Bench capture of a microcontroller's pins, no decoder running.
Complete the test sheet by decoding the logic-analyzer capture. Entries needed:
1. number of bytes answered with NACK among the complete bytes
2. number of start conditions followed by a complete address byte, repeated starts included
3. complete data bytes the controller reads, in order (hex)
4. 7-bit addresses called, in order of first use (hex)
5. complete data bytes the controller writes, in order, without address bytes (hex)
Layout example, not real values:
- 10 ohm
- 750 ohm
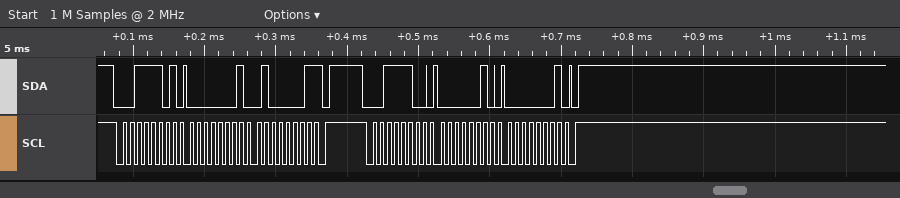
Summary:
- 1
- 2
- 01 41
- 0x1E
- 02 01
